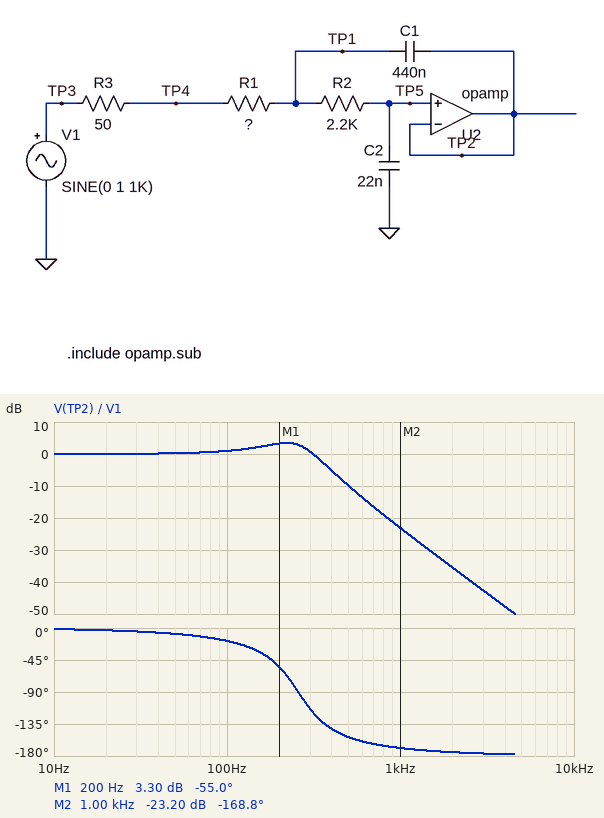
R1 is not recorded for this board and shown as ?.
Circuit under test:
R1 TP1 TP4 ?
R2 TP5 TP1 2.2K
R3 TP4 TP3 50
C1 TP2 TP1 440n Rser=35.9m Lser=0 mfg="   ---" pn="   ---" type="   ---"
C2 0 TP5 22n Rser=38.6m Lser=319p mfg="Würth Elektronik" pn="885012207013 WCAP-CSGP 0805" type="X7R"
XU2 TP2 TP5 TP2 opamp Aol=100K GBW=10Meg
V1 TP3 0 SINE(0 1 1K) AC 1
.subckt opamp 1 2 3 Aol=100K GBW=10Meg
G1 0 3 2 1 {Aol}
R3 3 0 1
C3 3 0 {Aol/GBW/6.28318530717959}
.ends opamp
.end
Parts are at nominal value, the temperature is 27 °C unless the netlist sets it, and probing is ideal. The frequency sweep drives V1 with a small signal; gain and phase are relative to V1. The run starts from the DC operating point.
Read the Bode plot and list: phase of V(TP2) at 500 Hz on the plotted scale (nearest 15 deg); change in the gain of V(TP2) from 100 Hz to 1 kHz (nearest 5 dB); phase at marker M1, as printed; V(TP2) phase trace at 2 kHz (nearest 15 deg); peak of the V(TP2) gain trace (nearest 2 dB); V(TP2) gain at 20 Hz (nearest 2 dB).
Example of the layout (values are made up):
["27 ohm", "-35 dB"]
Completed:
["-150 deg", "-25 dB", "-55.0 deg", "-180 deg", "4 dB", "0 dB"]
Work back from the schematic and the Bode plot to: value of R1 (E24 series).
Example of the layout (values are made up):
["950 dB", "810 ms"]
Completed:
["18 kΩ"]
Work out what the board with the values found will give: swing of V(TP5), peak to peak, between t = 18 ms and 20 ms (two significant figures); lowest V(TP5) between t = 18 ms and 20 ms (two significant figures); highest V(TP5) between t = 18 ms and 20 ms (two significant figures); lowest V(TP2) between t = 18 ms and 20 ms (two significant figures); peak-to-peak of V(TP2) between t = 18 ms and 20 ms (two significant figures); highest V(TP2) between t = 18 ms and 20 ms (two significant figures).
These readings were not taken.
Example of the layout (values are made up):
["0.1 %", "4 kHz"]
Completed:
["140 mV", "-69 mV", "69 mV", "-69 mV", "140 mV", "69 mV"]
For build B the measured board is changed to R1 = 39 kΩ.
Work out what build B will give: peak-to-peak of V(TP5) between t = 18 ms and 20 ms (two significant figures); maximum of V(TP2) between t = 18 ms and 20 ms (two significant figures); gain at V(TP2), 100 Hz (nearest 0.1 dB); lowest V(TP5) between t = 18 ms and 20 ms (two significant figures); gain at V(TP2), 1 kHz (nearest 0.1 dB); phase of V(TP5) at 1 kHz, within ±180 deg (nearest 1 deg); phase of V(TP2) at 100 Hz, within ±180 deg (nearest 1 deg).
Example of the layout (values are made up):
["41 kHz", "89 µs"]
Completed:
["62 mV", "31 mV", "1.1 dB", "-31 mV", "-30.2 dB", "-170 deg", "-40 deg"]
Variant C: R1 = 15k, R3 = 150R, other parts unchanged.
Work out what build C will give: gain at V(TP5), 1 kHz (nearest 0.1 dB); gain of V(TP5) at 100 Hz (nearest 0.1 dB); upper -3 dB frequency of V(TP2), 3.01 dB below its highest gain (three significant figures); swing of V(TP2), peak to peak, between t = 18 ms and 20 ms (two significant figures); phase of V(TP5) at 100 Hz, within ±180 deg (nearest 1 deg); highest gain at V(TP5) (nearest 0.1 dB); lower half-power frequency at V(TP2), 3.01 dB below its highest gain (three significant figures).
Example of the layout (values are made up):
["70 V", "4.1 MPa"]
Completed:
["-21.6 dB", "0.9 dB", "332 Hz", "170 mV", "-15 deg", "4.0 dB", "105 Hz"]
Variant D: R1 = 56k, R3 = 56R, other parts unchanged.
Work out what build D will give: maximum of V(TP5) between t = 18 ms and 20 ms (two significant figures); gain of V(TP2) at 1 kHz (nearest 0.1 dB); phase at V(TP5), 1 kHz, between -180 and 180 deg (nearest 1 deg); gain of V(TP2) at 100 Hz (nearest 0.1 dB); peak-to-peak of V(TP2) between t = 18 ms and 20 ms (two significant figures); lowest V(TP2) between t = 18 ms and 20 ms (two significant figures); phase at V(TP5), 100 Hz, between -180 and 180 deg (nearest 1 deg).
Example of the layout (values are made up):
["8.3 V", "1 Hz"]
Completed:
["21 mV", "-33.4 dB", "-170 deg", "0.3 dB", "43 mV", "-21 mV", "-57 deg"]
